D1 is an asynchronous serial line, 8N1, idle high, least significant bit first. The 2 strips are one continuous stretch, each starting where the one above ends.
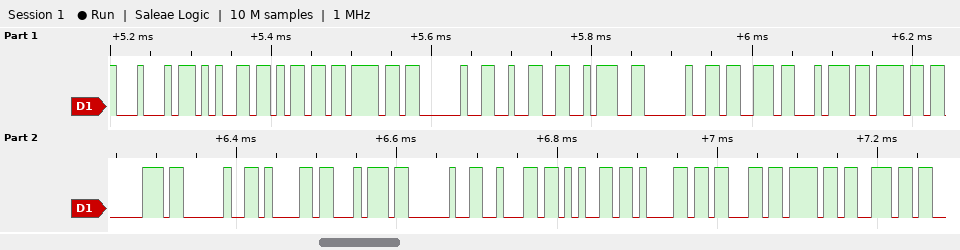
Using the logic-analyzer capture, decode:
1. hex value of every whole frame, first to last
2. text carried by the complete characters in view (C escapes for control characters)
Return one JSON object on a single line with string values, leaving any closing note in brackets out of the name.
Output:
{"hex value of every whole frame, first to last": "44 65 6D 6F 20 32 3A 20 73 74 6F 70 20 61 74 20 62 65 61 63 6F 6E", "text carried by the complete characters in view": "\"Demo 2: stop at beacon\""}
